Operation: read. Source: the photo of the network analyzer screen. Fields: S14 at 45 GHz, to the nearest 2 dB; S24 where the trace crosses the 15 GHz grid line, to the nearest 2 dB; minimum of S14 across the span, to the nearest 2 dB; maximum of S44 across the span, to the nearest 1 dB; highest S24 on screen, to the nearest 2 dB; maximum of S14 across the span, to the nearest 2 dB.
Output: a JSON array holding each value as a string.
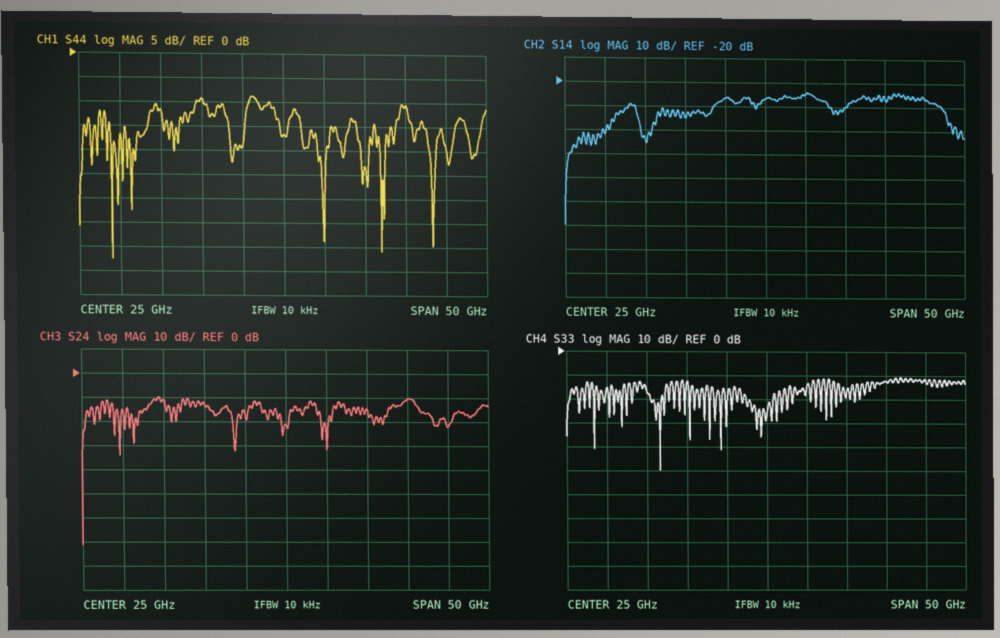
["-26 dB", "-12 dB", "-80 dB", "-9 dB", "-10 dB", "-24 dB"]
